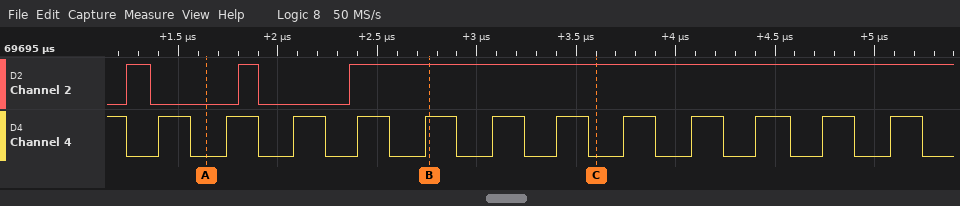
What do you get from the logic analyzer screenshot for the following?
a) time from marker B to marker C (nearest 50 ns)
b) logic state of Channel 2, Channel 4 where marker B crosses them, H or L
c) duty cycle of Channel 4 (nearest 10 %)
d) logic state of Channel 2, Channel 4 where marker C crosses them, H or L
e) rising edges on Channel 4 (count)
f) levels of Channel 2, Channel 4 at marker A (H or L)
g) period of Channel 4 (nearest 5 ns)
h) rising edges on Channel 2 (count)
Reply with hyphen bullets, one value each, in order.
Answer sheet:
- 850 ns
- Channel 2=H, Channel 4=H
- 50 %
- Channel 2=H, Channel 4=L
- 12
- Channel 2=L, Channel 4=L
- 335 ns
- 3
